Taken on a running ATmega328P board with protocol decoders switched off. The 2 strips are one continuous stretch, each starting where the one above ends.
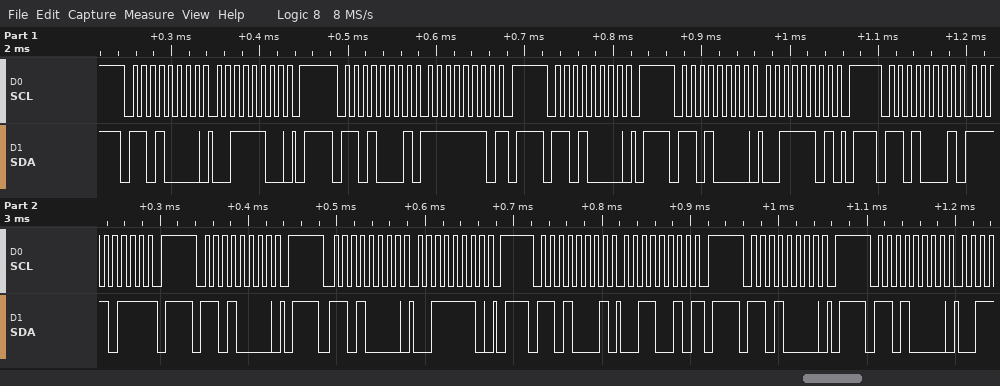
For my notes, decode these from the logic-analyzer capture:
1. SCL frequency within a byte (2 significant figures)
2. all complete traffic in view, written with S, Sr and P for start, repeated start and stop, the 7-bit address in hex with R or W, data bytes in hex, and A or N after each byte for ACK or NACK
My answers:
100 kHz
S 68W A 3C A P S 68R A FE N P S 68W A P S 68W A 3D A P S 68R A F7 N P S 68W A P S 68W A 3E A P S 68R A 32 N P S 68W A P S 68W A
